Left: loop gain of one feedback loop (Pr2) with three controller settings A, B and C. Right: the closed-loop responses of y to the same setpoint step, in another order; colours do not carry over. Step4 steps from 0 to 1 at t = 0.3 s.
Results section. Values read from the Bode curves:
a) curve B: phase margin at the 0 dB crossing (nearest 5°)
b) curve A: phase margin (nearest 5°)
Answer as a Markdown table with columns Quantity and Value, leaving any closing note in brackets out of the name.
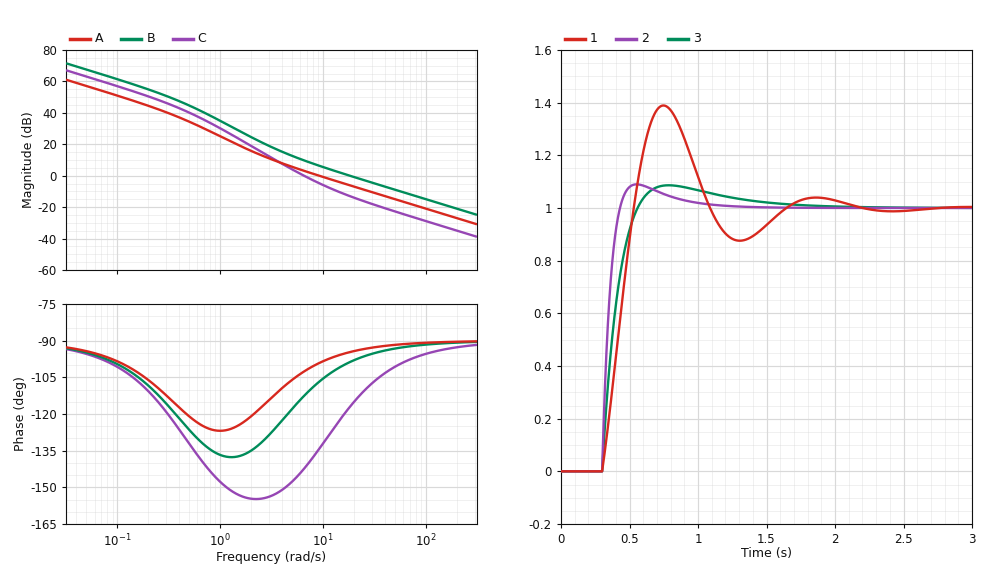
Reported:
| Quantity | Value |
|---|---|
| curve B: phase margin at the 0 dB crossing | 80° |
| curve A: phase margin | 80° |
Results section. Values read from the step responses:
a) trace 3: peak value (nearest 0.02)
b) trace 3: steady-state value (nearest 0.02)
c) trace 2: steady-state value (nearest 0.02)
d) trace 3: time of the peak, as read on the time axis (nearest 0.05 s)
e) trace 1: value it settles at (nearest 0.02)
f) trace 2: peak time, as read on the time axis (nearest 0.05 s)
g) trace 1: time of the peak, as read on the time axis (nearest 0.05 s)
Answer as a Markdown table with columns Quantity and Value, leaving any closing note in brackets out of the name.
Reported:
| Quantity | Value |
|---|---|
| trace 3: peak value | 1.08 |
| trace 3: steady-state value | 1.00 |
| trace 2: steady-state value | 1.00 |
| trace 3: time of the peak, as read on the time axis | 0.80 s |
| trace 1: value it settles at | 1.00 |
| trace 2: peak time, as read on the time axis | 0.55 s |
| trace 1: time of the peak, as read on the time axis | 0.75 s |
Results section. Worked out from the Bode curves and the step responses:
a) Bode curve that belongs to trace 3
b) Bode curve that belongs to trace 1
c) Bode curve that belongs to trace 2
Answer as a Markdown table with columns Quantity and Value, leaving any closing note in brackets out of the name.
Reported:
| Quantity | Value |
|---|---|
| Bode curve that belongs to trace 3 | A |
| Bode curve that belongs to trace 1 | C |
| Bode curve that belongs to trace 2 | B |
